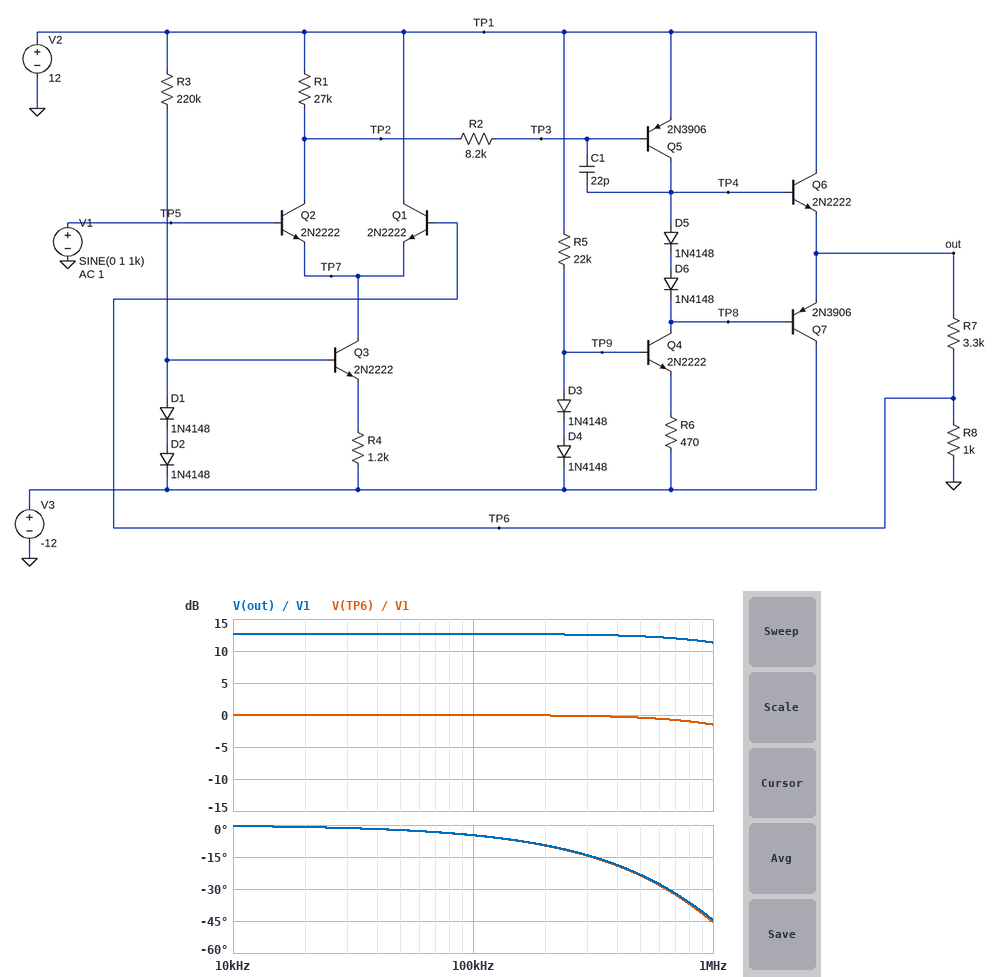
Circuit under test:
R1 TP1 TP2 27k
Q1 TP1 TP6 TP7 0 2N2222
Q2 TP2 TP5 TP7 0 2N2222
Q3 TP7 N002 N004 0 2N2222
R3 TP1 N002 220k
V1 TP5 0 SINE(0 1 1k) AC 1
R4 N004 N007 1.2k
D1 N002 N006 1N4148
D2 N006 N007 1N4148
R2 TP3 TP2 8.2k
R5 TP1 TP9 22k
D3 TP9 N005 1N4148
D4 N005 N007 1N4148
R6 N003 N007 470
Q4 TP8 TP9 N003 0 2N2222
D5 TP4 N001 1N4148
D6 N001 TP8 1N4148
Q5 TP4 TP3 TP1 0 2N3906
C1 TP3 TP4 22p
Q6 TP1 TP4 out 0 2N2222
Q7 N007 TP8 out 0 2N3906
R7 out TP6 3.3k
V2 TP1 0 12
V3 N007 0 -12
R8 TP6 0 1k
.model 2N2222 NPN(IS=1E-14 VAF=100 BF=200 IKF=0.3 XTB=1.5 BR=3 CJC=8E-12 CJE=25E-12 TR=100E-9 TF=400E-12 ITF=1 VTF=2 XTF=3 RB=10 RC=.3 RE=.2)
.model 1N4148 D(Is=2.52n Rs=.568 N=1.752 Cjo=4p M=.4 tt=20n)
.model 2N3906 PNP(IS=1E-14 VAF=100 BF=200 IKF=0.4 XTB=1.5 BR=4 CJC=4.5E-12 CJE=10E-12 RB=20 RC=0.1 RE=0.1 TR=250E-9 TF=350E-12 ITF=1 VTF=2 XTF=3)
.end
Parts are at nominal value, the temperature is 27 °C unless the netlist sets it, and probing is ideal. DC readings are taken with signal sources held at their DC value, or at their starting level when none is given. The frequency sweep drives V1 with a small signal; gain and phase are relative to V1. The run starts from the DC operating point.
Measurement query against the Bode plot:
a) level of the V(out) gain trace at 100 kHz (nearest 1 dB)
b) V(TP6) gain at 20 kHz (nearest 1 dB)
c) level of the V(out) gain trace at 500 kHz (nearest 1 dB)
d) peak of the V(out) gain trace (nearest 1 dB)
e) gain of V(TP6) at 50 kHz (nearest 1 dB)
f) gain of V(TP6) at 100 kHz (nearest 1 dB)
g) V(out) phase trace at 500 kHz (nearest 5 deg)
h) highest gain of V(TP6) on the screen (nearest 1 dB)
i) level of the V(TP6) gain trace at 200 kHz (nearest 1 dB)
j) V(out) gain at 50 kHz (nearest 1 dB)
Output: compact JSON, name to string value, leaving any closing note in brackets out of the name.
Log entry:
{"level of the V(out) gain trace at 100 kHz": "13 dB", "V(TP6) gain at 20 kHz": "0 dB", "level of the V(out) gain trace at 500 kHz": "12 dB", "peak of the V(out) gain trace": "13 dB", "gain of V(TP6) at 50 kHz": "0 dB", "gain of V(TP6) at 100 kHz": "0 dB", "V(out) phase trace at 500 kHz": "-25 deg", "highest gain of V(TP6) on the screen": "0 dB", "level of the V(TP6) gain trace at 200 kHz": "0 dB", "V(out) gain at 50 kHz": "13 dB"}
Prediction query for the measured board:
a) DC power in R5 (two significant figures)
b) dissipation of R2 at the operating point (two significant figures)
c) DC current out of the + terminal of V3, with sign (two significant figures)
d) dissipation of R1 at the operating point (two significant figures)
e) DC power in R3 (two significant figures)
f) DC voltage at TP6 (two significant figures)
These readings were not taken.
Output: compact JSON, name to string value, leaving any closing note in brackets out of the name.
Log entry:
{"DC power in R5": "24 mW", "dissipation of R2 at the operating point": "200 nW", "DC current out of the + terminal of V3, with sign": "-2.6 mA", "dissipation of R1 at the operating point": "18 µW", "DC power in R3": "2.4 mW", "DC voltage at TP6": "54 mV"}
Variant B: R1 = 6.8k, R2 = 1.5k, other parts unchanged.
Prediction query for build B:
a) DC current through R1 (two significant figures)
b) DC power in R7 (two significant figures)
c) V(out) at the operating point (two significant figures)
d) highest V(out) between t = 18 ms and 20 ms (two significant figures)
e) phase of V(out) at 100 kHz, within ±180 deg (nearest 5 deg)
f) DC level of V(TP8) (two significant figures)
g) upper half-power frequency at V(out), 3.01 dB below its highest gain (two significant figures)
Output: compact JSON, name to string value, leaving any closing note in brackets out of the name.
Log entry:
{"DC current through R1": "97 µA", "DC power in R7": "780 nW", "V(out) at the operating point": "65 mV", "highest V(out) between t = 18 ms and 20 ms": "4.4 V", "phase of V(out) at 100 kHz, within ±180 deg": "0 deg", "DC level of V(TP8)": "-520 mV", "upper half-power frequency at V(out), 3.01 dB below its highest gain": "5.0 MHz"}
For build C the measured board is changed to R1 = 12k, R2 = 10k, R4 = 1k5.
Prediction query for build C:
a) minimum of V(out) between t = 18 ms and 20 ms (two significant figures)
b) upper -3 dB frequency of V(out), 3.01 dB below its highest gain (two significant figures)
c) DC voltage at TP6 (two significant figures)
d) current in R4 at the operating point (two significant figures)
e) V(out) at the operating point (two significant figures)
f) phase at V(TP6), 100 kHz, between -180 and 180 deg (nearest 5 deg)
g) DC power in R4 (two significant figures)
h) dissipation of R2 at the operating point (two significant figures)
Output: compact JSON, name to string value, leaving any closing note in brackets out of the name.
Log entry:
{"minimum of V(out) between t = 18 ms and 20 ms": "-4.2 V", "upper -3 dB frequency of V(out), 3.01 dB below its highest gain": "2.1 MHz", "DC voltage at TP6": "25 mV", "current in R4 at the operating point": "230 µA", "V(out) at the operating point": "110 mV", "phase at V(TP6), 100 kHz, between -180 and 180 deg": "-5 deg", "DC power in R4": "81 µW", "dissipation of R2 at the operating point": "250 nW"}
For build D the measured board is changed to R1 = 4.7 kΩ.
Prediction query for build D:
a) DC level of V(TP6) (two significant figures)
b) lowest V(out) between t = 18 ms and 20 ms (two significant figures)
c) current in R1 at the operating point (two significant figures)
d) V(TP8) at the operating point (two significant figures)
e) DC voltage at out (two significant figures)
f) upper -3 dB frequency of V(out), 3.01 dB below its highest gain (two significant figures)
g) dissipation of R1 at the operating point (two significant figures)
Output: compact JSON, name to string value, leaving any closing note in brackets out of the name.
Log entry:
{"DC level of V(TP6)": "-4.4 mV", "lowest V(out) between t = 18 ms and 20 ms": "-4.3 V", "current in R1 at the operating point": "150 µA", "V(TP8) at the operating point": "-610 mV", "DC voltage at out": "-17 mV", "upper -3 dB frequency of V(out), 3.01 dB below its highest gain": "2.0 MHz", "dissipation of R1 at the operating point": "100 µW"}
